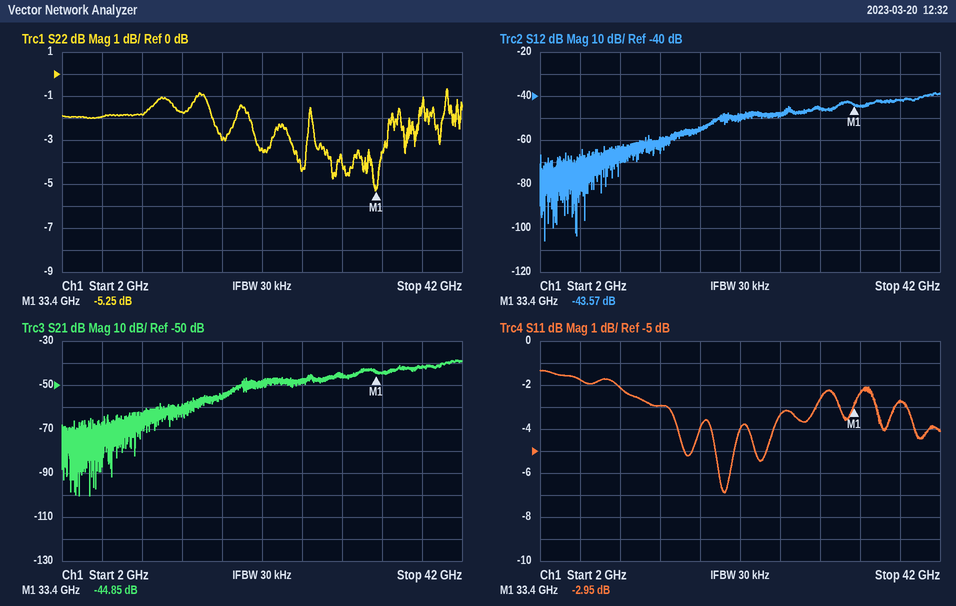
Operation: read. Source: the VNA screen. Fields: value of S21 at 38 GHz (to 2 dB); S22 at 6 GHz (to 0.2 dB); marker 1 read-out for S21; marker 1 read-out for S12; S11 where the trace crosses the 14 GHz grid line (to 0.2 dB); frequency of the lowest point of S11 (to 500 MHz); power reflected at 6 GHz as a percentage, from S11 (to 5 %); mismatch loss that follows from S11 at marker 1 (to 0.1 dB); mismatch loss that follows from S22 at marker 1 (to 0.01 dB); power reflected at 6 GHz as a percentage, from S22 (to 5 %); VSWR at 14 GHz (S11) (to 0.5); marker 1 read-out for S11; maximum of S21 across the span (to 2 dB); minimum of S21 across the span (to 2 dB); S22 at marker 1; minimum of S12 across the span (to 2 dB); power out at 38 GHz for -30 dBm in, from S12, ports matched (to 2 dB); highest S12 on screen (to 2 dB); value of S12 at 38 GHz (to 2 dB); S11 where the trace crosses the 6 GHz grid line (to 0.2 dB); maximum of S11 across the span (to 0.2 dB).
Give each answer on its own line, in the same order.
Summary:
-42 dB
-2.0 dB
-44.85 dB
-43.57 dB
-3.0 dB
20.5 GHz
65 %
3.1 dB
1.54 dB
65 %
6.0
-2.95 dB
-38 dB
-100 dB
-5.25 dB
-106 dB
-72 dBm
-38 dB
-42 dB
-1.8 dB
-1.4 dB
